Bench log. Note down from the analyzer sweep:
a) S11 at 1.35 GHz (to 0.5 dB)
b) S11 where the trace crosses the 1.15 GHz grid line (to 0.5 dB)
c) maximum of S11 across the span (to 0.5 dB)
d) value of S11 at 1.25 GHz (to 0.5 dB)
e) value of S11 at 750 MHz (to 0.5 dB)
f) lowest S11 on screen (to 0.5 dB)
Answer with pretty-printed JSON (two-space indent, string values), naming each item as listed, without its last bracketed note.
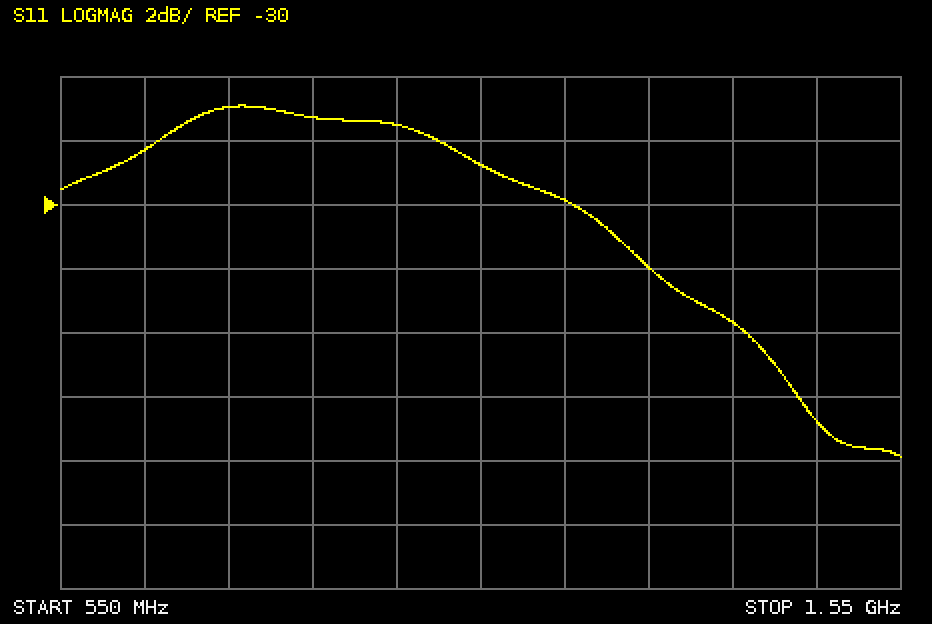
{
  "S11 at 1.35 GHz": "-33.5 dB",
  "S11 where the trace crosses the 1.15 GHz grid line": "-30.0 dB",
  "maximum of S11 across the span": "-27.0 dB",
  "value of S11 at 1.25 GHz": "-32.0 dB",
  "value of S11 at 750 MHz": "-27.0 dB",
  "lowest S11 on screen": "-38.0 dB"
}
